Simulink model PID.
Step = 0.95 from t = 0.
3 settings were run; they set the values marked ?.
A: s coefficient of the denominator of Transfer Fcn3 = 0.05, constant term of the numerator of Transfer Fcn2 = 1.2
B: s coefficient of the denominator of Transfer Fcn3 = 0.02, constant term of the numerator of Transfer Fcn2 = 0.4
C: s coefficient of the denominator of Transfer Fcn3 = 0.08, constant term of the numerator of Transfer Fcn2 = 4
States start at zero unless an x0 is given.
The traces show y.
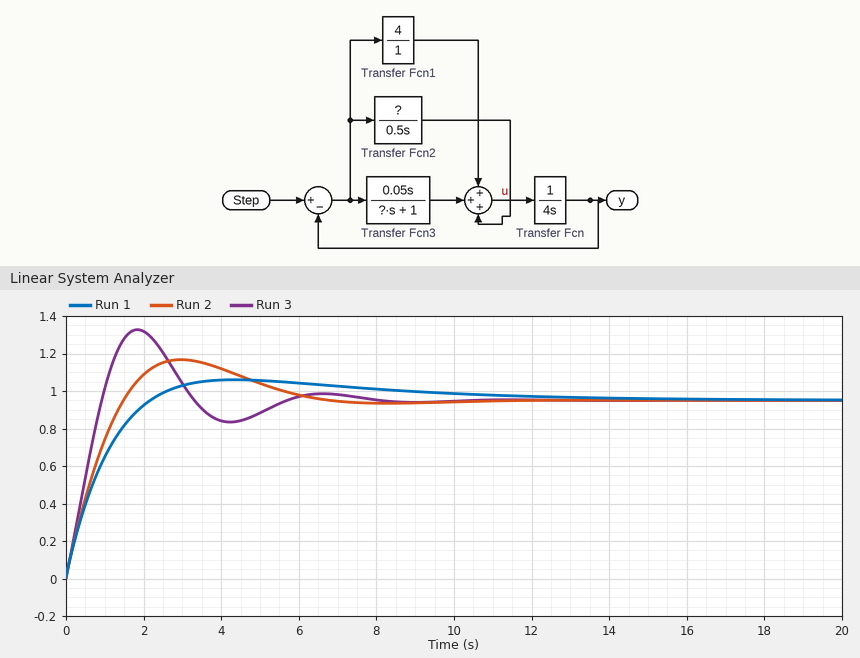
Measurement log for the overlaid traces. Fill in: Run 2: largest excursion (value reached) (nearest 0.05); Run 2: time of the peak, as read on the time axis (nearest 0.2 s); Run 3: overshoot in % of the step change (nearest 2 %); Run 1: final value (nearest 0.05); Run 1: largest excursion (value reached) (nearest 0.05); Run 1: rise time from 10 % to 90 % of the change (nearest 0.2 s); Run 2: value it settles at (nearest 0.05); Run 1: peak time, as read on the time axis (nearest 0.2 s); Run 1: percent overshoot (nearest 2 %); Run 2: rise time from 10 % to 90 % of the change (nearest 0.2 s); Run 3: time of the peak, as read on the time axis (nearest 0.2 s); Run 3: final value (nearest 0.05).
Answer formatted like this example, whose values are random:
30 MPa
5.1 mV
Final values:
1.15
3.0 s
40 %
0.95
1.05
1.6 s
0.95
4.4 s
12 %
1.2 s
1.8 s
0.95
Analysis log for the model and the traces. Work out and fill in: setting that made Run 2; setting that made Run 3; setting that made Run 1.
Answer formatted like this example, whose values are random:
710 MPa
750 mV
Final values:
A
C
B
